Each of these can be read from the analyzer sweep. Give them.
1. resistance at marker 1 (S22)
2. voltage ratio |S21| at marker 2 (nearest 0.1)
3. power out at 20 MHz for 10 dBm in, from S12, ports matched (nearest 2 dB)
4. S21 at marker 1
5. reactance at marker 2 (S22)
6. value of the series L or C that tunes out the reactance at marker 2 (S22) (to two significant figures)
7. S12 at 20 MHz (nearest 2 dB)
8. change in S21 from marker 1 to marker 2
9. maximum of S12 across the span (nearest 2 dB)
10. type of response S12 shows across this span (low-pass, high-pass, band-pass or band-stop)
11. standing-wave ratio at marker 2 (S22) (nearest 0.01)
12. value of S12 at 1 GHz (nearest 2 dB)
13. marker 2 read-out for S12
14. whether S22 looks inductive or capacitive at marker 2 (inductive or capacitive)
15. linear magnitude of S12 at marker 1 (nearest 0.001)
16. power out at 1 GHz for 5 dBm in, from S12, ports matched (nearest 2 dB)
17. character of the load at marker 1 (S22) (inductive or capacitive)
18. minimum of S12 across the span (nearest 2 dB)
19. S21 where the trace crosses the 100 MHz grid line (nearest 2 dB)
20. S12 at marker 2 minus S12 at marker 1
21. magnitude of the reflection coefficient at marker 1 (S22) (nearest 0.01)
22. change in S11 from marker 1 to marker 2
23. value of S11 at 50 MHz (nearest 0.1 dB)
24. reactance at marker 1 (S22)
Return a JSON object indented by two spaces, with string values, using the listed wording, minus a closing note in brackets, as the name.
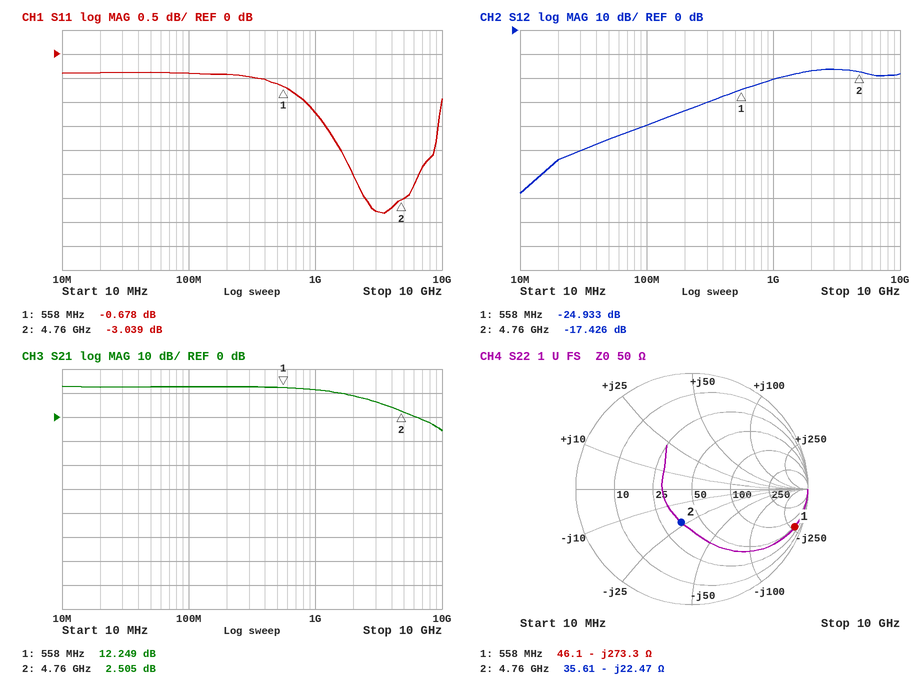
{
  "resistance at marker 1": "46.1 Ω",
  "voltage ratio |S21| at marker 2": "1.3",
  "power out at 20 MHz for 10 dBm in, from S12, ports matched": "-44 dBm",
  "S21 at marker 1": "12.249 dB",
  "reactance at marker 2": "-22.47 Ω",
  "value of the series L or C that tunes out the reactance at marker 2 (S22)": "750 pH",
  "S12 at 20 MHz": "-54 dB",
  "change in S21 from marker 1 to marker 2": "-9.744 dB",
  "maximum of S12 across the span": "-16 dB",
  "type of response S12 shows across this span": "high-pass",
  "standing-wave ratio at marker 2 (S22)": "1.86",
  "value of S12 at 1 GHz": "-20 dB",
  "marker 2 read-out for S12": "-17.426 dB",
  "whether S22 looks inductive or capacitive at marker 2": "capacitive",
  "linear magnitude of S12 at marker 1": "0.057",
  "power out at 1 GHz for 5 dBm in, from S12, ports matched": "-16 dBm",
  "character of the load at marker 1 (S22)": "capacitive",
  "minimum of S12 across the span": "-68 dB",
  "S21 where the trace crosses the 100 MHz grid line": "12 dB",
  "S12 at marker 2 minus S12 at marker 1": "7.507 dB",
  "magnitude of the reflection coefficient at marker 1 (S22)": "0.94",
  "change in S11 from marker 1 to marker 2": "-2.361 dB",
  "value of S11 at 50 MHz": "-0.4 dB",
  "reactance at marker 1": "-273.3 Ω"
}
